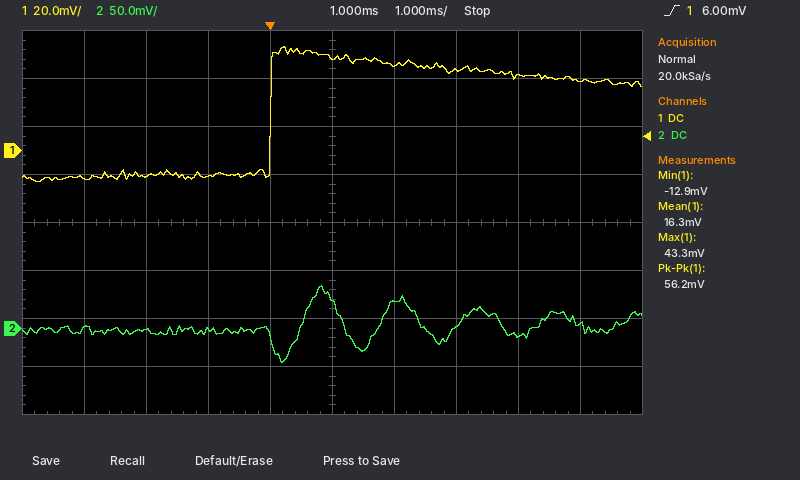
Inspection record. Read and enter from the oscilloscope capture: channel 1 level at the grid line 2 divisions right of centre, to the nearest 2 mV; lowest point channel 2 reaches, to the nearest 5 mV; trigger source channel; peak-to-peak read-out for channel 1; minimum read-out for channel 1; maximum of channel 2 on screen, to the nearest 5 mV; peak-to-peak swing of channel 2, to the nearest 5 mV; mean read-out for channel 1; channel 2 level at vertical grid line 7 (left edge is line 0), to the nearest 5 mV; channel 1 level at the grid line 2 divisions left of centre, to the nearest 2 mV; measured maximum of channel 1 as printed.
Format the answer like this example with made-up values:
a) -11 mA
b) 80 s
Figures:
a) 34 mV
b) -35 mV
c) channel 1
d) 56.2 mV
e) -12.9 mV
f) 45 mV
g) 80 mV
h) 16.3 mV
i) 0 mV
j) -10 mV
k) 43.3 mV
